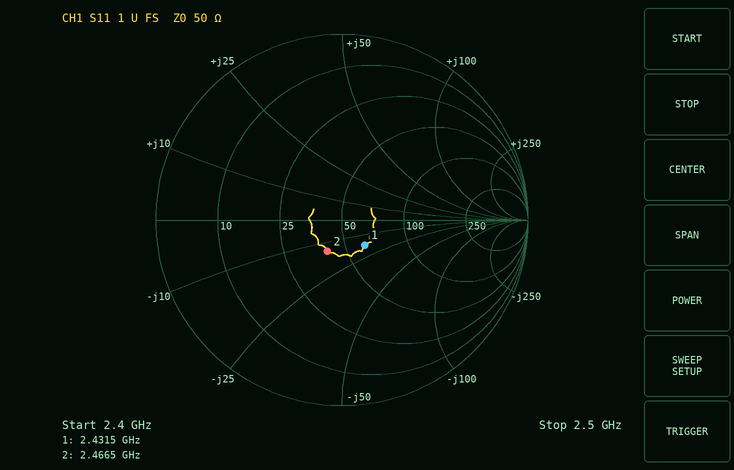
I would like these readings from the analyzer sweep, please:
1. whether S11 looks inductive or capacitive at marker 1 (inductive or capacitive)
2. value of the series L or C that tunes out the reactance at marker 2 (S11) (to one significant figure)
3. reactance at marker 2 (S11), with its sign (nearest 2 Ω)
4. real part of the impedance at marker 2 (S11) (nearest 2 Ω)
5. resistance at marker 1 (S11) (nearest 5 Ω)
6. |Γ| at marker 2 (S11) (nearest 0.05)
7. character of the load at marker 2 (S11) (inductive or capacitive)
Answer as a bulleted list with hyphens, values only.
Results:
- capacitive
- 900 pH
- -14 Ω
- 40 Ω
- 60 Ω
- 0.20
- capacitive
